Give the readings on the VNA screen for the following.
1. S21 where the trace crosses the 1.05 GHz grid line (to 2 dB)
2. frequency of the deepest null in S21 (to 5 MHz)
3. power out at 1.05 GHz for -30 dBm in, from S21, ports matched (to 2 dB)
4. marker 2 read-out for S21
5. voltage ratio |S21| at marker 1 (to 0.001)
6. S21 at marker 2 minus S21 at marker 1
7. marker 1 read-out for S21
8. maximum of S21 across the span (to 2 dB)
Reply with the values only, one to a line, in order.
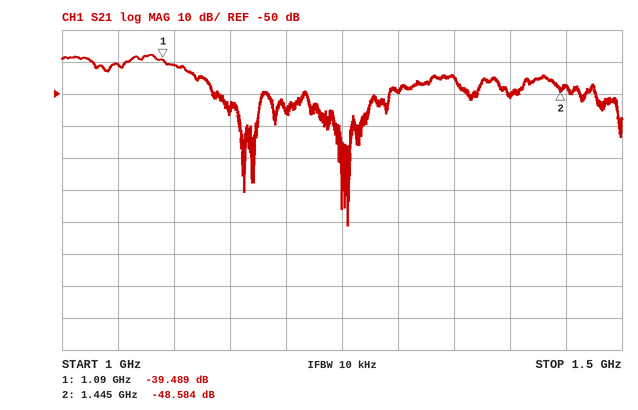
-40 dB
1.255 GHz
-70 dBm
-48.584 dB
0.011
-9.095 dB
-39.489 dB
-38 dB
